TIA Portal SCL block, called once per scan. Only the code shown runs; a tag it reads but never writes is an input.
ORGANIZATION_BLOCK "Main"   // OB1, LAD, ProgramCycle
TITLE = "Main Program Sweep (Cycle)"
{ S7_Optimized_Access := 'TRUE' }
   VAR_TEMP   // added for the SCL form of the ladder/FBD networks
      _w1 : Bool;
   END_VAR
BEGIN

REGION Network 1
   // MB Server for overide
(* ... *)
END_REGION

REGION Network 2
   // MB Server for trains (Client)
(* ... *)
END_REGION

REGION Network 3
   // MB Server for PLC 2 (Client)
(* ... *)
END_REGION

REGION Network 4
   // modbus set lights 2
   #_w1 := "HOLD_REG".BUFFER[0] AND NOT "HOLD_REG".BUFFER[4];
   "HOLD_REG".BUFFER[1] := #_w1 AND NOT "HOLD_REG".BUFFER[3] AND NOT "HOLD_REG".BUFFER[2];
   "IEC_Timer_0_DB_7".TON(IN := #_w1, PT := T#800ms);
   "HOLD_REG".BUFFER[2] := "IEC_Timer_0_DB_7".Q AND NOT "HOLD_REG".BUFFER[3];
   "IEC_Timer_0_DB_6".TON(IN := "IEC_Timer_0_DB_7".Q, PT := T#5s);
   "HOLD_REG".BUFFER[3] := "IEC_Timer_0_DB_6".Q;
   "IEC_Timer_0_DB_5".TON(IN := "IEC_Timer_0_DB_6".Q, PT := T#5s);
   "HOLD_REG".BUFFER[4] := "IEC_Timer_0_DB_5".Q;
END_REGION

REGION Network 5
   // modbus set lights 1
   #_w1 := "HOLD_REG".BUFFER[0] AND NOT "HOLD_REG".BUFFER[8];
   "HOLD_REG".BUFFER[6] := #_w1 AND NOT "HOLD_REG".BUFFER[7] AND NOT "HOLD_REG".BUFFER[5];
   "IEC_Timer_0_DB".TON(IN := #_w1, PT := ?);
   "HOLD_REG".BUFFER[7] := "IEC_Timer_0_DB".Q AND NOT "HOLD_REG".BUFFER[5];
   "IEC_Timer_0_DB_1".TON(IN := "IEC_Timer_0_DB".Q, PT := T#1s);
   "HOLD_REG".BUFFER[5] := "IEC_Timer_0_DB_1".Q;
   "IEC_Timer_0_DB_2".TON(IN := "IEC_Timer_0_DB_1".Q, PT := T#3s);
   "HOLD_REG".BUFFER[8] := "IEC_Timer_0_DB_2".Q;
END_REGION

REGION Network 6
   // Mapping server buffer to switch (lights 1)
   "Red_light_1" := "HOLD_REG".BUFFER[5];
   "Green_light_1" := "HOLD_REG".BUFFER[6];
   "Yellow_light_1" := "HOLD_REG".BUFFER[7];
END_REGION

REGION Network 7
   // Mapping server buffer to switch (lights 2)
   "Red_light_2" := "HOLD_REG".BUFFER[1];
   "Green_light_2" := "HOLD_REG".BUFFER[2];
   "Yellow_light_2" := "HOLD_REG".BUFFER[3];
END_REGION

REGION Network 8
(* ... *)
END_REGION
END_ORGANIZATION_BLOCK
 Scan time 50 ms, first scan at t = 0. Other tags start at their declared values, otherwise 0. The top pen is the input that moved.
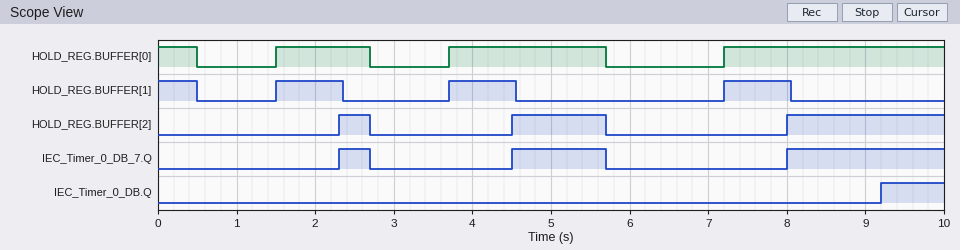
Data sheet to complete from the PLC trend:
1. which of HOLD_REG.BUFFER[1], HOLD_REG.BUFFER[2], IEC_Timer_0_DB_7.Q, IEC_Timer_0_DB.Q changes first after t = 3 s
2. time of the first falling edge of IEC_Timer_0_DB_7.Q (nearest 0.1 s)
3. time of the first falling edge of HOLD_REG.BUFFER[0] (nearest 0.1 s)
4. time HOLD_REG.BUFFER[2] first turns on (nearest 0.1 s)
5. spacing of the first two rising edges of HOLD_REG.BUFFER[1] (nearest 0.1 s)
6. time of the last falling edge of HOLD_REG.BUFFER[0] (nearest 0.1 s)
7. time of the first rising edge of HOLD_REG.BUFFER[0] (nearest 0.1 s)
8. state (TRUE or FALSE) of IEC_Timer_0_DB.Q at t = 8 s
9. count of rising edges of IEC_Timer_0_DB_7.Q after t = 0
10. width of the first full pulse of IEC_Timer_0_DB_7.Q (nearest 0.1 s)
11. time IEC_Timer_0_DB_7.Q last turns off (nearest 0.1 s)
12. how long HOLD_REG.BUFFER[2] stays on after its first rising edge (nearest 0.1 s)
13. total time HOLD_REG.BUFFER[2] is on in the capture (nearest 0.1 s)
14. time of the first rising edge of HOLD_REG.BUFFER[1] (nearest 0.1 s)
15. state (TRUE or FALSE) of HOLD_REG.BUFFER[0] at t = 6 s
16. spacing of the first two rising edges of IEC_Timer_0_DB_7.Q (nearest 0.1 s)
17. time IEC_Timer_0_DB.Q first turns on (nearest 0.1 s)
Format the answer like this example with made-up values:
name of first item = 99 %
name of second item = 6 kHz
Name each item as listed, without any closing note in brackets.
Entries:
which of HOLD_REG.BUFFER[1], HOLD_REG.BUFFER[2], IEC_Timer_0_DB_7.Q, IEC_Timer_0_DB.Q changes first after t = 3 s = HOLD_REG.BUFFER[1]
time of the first falling edge of IEC_Timer_0_DB_7.Q = 2.7 s
time of the first falling edge of HOLD_REG.BUFFER[0] = 0.5 s
time HOLD_REG.BUFFER[2] first turns on = 2.3 s
spacing of the first two rising edges of HOLD_REG.BUFFER[1] = 2.2 s
time of the last falling edge of HOLD_REG.BUFFER[0] = 5.7 s
time of the first rising edge of HOLD_REG.BUFFER[0] = 1.5 s
state (TRUE or FALSE) of IEC_Timer_0_DB.Q at t = 8 s = FALSE
count of rising edges of IEC_Timer_0_DB_7.Q after t = 0 = 3
width of the first full pulse of IEC_Timer_0_DB_7.Q = 0.4 s
time IEC_Timer_0_DB_7.Q last turns off = 5.7 s
how long HOLD_REG.BUFFER[2] stays on after its first rising edge = 0.4 s
total time HOLD_REG.BUFFER[2] is on in the capture = 3.6 s
time of the first rising edge of HOLD_REG.BUFFER[1] = 1.5 s
state (TRUE or FALSE) of HOLD_REG.BUFFER[0] at t = 6 s = FALSE
spacing of the first two rising edges of IEC_Timer_0_DB_7.Q = 2.2 s
time IEC_Timer_0_DB.Q first turns on = 9.2 s
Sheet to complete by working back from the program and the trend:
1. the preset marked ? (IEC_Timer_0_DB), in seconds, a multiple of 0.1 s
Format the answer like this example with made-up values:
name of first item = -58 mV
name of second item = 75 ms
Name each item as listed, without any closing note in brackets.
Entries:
the preset marked ? (IEC_Timer_0_DB), in seconds, a multiple of 0.1 s = 2.0 s
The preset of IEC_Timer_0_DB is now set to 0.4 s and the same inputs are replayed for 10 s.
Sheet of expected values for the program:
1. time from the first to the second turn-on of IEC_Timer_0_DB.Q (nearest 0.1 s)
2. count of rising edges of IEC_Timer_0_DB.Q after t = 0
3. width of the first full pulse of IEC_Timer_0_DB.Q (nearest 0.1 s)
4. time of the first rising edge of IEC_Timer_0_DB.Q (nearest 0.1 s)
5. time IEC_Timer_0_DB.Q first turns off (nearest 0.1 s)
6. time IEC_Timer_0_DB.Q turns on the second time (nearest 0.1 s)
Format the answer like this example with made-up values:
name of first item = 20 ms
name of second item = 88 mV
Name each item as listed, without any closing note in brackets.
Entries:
time from the first to the second turn-on of IEC_Timer_0_DB.Q = 1.5 s
count of rising edges of IEC_Timer_0_DB.Q after t = 0 = 4
width of the first full pulse of IEC_Timer_0_DB.Q = 0.1 s
time of the first rising edge of IEC_Timer_0_DB.Q = 0.4 s
time IEC_Timer_0_DB.Q first turns off = 0.5 s
time IEC_Timer_0_DB.Q turns on the second time = 1.9 s
